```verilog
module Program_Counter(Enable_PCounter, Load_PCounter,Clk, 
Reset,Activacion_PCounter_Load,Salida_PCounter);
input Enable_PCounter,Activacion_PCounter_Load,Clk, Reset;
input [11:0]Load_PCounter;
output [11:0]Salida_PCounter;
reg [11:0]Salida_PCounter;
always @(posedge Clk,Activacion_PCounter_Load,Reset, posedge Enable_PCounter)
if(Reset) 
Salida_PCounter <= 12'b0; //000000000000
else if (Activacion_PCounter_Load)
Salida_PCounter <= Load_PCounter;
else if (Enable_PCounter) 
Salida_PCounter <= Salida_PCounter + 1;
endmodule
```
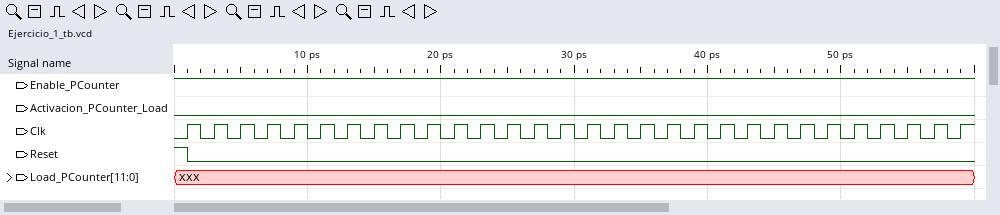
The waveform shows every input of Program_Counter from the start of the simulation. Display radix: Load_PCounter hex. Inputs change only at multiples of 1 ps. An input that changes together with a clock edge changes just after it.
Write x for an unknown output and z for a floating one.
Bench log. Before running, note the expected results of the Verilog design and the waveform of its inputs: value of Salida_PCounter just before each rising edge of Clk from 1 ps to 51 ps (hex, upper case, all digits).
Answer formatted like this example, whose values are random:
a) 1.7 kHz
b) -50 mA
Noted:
a) 000, 001, 002, 003, 004, 005, 006, 007, 008, 009, 00A, 00B, 00C, 00D, 00E, 00F, 010, 011, 012, 013, 014, 015, 016, 017, 018, 019
